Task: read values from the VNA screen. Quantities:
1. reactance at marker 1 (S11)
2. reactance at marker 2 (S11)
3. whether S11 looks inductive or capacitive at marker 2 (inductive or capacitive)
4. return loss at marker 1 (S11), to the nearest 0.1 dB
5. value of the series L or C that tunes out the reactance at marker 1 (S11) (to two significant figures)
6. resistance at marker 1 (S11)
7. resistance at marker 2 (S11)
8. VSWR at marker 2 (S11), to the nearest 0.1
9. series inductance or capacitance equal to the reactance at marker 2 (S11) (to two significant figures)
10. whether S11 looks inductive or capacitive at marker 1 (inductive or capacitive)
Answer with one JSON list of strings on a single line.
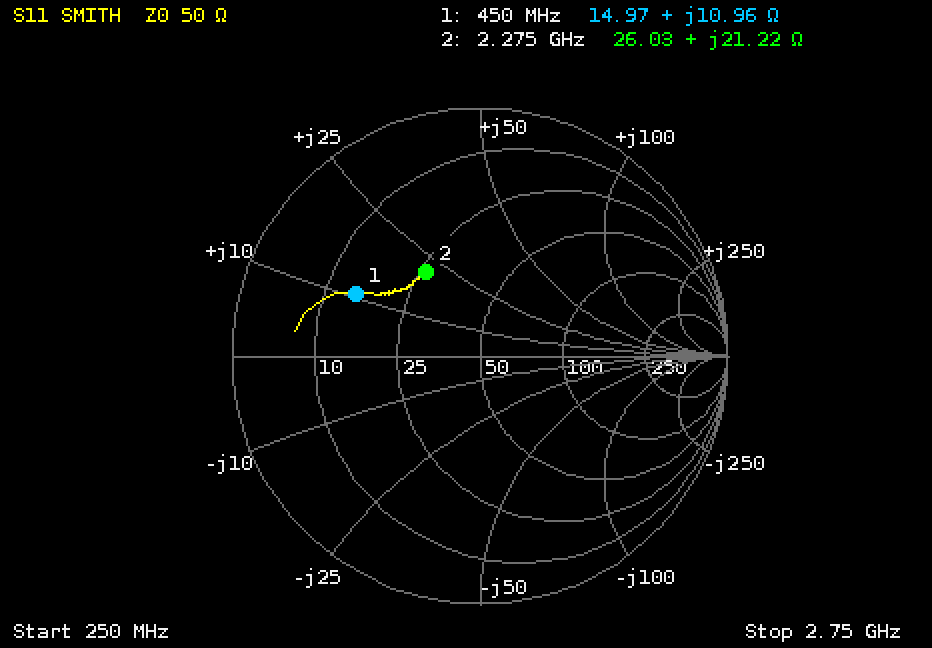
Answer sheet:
["+10.96 Ω", "+21.22 Ω", "inductive", "5.1 dB", "32 pF", "14.97 Ω", "26.03 Ω", "2.4", "1.5 nH", "inductive"]
